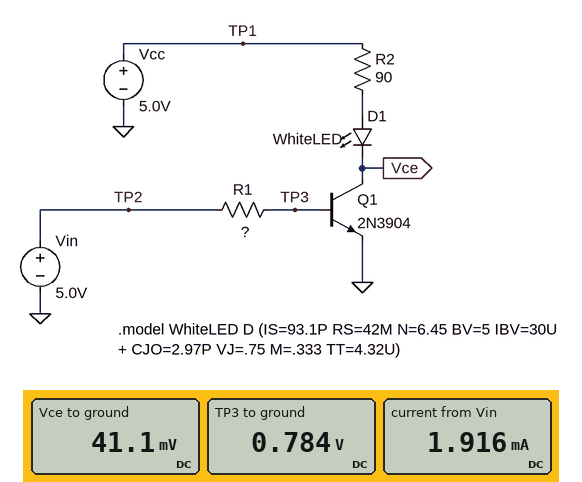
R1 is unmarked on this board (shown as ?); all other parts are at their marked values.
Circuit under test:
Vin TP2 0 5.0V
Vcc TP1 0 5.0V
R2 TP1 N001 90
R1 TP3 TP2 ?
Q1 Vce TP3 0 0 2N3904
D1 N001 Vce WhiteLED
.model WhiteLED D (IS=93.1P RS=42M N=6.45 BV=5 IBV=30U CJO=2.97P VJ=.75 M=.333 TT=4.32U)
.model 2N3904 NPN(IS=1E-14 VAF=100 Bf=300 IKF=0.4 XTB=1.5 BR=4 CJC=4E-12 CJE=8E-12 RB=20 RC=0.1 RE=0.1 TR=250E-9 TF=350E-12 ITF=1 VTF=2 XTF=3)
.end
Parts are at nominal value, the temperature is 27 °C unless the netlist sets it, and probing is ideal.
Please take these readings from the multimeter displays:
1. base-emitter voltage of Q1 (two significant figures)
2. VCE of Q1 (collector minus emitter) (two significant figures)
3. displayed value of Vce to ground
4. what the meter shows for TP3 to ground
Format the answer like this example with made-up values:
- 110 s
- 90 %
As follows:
- 780 mV
- 41 mV
- 41.1 mV
- 0.784 V
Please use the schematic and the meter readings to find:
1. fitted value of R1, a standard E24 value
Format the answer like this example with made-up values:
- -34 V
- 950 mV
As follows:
- 2.2 kΩ
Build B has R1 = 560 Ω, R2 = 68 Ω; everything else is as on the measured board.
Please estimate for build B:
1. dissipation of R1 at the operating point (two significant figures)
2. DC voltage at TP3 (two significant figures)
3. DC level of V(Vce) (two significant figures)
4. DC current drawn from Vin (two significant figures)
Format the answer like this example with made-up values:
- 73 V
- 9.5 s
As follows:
- 30 mW
- 910 mV
- 28 mV
- 7.3 mA
